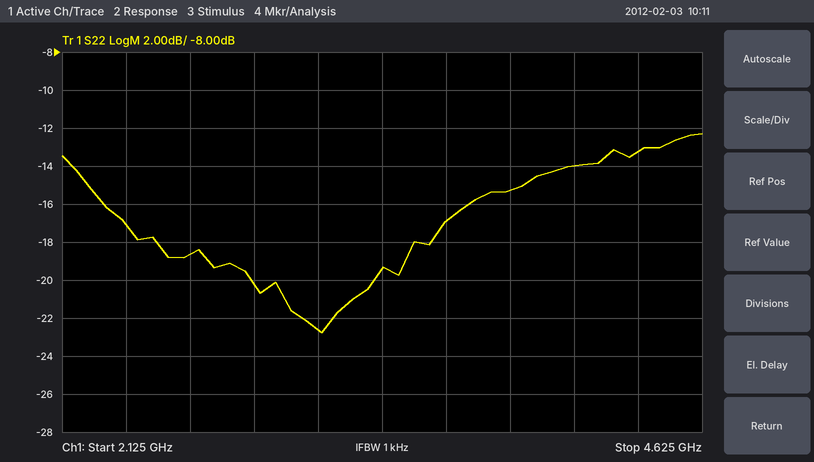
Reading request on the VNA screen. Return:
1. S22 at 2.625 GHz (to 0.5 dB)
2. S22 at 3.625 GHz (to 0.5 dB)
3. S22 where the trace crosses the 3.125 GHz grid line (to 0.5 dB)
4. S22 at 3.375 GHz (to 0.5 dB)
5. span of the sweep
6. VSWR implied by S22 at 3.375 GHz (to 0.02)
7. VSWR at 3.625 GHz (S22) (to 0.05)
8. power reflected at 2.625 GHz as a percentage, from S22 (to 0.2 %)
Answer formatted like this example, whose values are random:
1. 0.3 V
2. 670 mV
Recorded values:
1. -18.5 dB
2. -17.0 dB
3. -22.5 dB
4. -19.5 dB
5. 2.5 GHz
6. 1.24
7. 1.35
8. 1.4 %
